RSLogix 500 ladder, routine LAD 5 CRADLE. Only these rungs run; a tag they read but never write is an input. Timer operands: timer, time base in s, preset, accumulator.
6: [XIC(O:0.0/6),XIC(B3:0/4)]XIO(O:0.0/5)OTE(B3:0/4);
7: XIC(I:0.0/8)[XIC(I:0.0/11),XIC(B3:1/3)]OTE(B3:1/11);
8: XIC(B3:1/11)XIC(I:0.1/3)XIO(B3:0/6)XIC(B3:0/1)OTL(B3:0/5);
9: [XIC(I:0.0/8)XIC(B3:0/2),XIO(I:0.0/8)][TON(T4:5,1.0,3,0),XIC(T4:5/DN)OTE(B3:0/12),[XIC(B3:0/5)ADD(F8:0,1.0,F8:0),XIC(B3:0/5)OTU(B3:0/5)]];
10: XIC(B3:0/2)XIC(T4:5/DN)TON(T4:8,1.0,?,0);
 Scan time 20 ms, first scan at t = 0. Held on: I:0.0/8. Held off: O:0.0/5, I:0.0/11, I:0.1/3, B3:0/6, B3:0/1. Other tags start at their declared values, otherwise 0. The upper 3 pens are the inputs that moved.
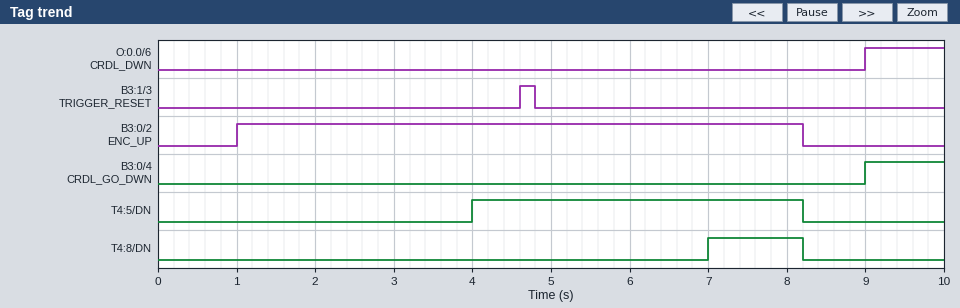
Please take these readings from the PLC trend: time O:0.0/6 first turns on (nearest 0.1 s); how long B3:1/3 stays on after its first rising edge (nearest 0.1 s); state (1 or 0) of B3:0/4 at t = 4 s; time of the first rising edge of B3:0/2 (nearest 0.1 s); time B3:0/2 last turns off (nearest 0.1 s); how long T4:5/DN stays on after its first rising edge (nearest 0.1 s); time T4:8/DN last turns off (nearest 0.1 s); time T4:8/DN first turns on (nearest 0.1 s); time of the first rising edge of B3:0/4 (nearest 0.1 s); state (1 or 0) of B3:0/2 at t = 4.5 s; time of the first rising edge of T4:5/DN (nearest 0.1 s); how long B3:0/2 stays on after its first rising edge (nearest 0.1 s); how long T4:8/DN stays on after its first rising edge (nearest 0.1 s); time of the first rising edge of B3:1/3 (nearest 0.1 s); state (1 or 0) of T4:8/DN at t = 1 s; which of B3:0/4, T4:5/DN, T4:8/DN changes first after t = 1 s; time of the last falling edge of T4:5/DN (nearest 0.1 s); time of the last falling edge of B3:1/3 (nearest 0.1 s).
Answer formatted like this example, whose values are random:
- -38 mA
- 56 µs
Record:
- 9.0 s
- 0.2 s
- 0
- 1.0 s
- 8.2 s
- 4.2 s
- 8.2 s
- 7.0 s
- 9.0 s
- 1
- 4.0 s
- 7.2 s
- 1.2 s
- 4.6 s
- 0
- T4:5/DN
- 8.2 s
- 4.8 s
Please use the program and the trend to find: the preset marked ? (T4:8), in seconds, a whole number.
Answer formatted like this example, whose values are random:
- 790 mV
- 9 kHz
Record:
- 3 s
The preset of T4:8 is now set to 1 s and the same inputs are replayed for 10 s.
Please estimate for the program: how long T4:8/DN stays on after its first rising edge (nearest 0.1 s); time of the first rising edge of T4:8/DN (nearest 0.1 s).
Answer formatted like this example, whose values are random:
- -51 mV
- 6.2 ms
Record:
- 3.2 s
- 5.0 s
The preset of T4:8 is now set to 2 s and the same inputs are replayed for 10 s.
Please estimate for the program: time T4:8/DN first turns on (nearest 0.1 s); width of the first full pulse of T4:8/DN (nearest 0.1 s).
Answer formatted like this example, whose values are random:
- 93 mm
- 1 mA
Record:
- 6.0 s
- 2.2 s
